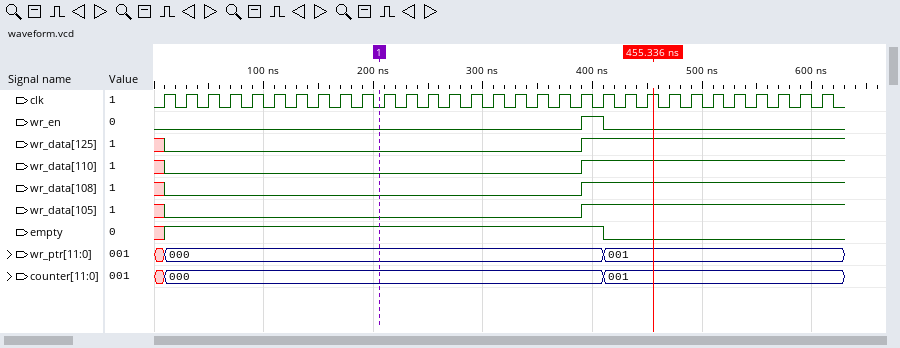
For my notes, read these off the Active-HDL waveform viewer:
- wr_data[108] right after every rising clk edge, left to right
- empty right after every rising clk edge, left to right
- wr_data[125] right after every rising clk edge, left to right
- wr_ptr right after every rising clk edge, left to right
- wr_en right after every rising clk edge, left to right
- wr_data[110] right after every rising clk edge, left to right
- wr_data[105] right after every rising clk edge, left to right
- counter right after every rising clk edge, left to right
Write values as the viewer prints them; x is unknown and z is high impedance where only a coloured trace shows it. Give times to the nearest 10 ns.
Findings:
0 0 0 0 0 0 0 0 0 0 0 0 0 0 0 0 0 0 0 1 1 1 1 1 1 1 1 1 1 1 1
1 1 1 1 1 1 1 1 1 1 1 1 1 1 1 1 1 1 1 1 0 0 0 0 0 0 0 0 0 0 0
0 0 0 0 0 0 0 0 0 0 0 0 0 0 0 0 0 0 0 1 1 1 1 1 1 1 1 1 1 1 1
000, 000, 000, 000, 000, 000, 000, 000, 000, 000, 000, 000, 000, 000, 000, 000, 000, 000, 000, 000, 001, 001, 001, 001, 001, 001, 001, 001, 001, 001, 001
0 0 0 0 0 0 0 0 0 0 0 0 0 0 0 0 0 0 0 1 0 0 0 0 0 0 0 0 0 0 0
0 0 0 0 0 0 0 0 0 0 0 0 0 0 0 0 0 0 0 1 1 1 1 1 1 1 1 1 1 1 1
0 0 0 0 0 0 0 0 0 0 0 0 0 0 0 0 0 0 0 1 1 1 1 1 1 1 1 1 1 1 1
000, 000, 000, 000, 000, 000, 000, 000, 000, 000, 000, 000, 000, 000, 000, 000, 000, 000, 000, 000, 001, 001, 001, 001, 001, 001, 001, 001, 001, 001, 001
